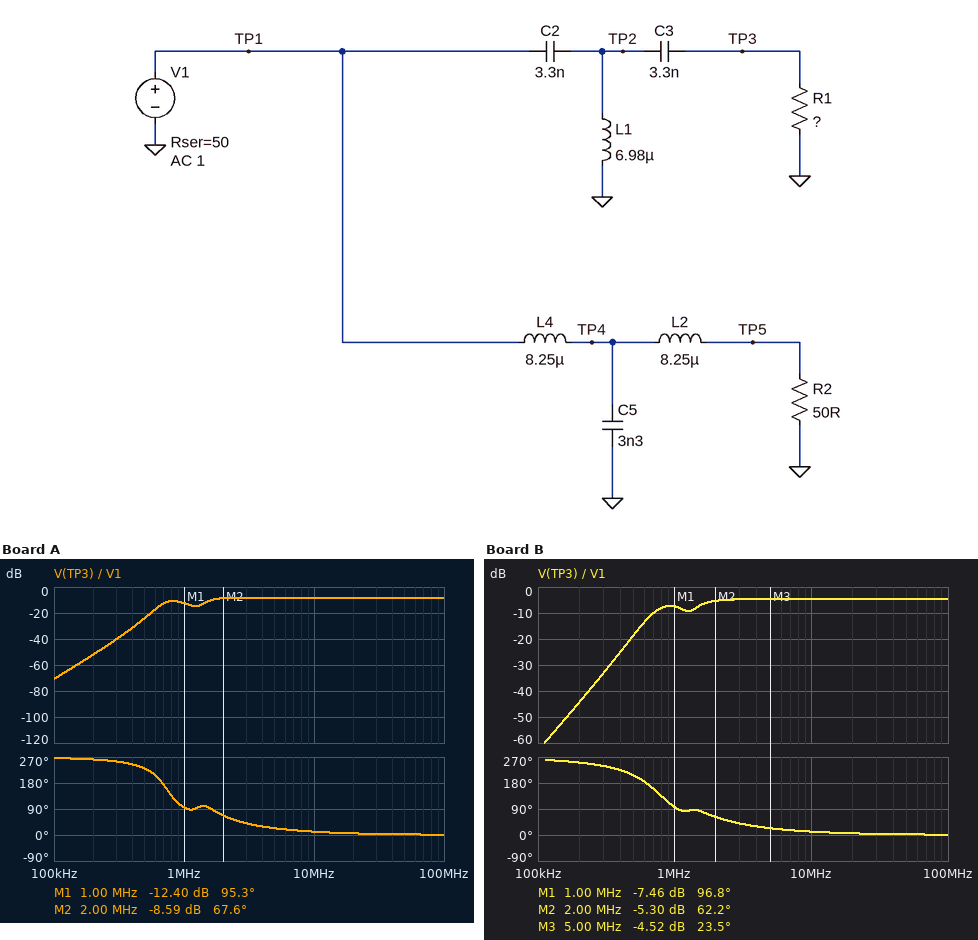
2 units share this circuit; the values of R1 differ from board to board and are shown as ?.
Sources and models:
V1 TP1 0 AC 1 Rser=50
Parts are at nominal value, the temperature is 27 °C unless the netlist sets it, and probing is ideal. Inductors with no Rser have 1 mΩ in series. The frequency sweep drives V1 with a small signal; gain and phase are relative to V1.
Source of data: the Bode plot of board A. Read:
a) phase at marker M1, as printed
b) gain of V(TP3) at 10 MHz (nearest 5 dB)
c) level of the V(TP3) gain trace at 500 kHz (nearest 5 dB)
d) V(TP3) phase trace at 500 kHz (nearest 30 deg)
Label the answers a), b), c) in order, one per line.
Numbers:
a) 95.3 deg
b) -10 dB
c) -25 dB
d) 240 deg
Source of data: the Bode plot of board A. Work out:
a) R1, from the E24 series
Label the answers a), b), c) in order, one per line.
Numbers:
a) 30 Ω
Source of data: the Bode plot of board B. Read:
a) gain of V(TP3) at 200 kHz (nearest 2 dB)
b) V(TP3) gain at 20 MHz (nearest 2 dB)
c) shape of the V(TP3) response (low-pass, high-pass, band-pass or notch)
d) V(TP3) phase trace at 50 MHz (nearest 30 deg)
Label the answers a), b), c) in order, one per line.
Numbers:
a) -44 dB
b) -4 dB
c) high-pass
d) 0 deg
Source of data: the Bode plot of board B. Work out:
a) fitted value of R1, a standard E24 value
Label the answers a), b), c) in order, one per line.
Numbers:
a) 75 Ω
